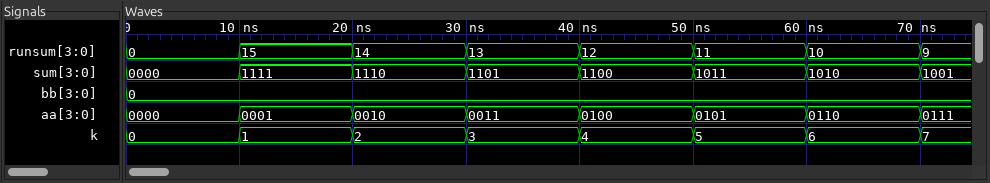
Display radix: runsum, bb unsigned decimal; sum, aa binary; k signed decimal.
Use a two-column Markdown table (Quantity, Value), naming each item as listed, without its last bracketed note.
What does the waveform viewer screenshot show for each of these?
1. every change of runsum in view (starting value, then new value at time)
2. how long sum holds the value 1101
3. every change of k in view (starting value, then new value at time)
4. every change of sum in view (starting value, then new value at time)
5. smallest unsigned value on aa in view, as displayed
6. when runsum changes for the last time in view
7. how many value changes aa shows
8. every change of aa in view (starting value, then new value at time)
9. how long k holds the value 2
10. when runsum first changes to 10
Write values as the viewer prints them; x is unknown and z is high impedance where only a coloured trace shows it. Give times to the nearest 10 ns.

| Quantity | Value |
|---|---|
| every change of runsum in view | 0, 15 at 10 ns, 14 at 20 ns, 13 at 30 ns, 12 at 40 ns, 11 at 50 ns, 10 at 60 ns, 9 at 70 ns |
| how long sum holds the value 1101 | 10 ns |
| every change of k in view | 0, 1 at 10 ns, 2 at 20 ns, 3 at 30 ns, 4 at 40 ns, 5 at 50 ns, 6 at 60 ns, 7 at 70 ns |
| every change of sum in view | 0000, 1111 at 10 ns, 1110 at 20 ns, 1101 at 30 ns, 1100 at 40 ns, 1011 at 50 ns, 1010 at 60 ns, 1001 at 70 ns |
| smallest unsigned value on aa in view, as displayed | 0000 |
| when runsum changes for the last time in view | 70 ns |
| how many value changes aa shows | 7 |
| every change of aa in view | 0000, 0001 at 10 ns, 0010 at 20 ns, 0011 at 30 ns, 0100 at 40 ns, 0101 at 50 ns, 0110 at 60 ns, 0111 at 70 ns |
| how long k holds the value 2 | 10 ns |
| when runsum first changes to 10 | 60 ns |
